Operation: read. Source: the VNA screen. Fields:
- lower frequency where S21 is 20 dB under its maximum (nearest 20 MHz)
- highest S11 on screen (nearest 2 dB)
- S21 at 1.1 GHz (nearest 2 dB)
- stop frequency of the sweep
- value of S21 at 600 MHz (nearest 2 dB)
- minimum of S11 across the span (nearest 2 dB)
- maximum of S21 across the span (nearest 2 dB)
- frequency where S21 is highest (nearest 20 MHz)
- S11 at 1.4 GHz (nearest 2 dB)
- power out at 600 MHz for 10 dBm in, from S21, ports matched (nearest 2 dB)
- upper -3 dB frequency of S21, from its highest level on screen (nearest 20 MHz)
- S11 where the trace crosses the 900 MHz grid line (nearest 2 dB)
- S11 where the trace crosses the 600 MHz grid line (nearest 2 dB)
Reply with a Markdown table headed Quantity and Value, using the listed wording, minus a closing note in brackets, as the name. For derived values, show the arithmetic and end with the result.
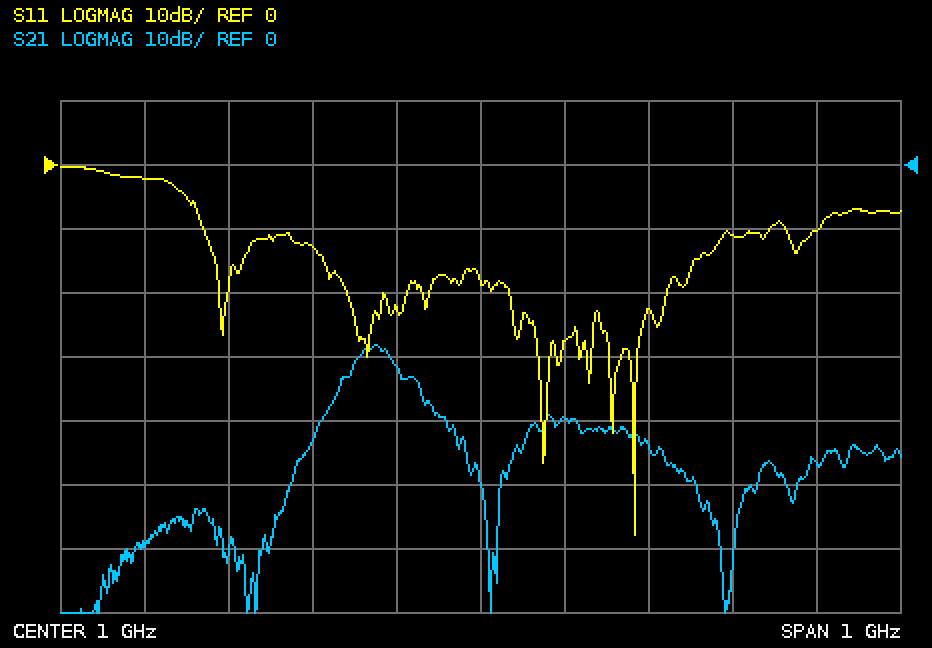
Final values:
| Quantity | Value |
|---|---|
| lower frequency where S21 is 20 dB under its maximum | 780 MHz |
| highest S11 on screen | 0 dB |
| S21 at 1.1 GHz | -40 dB |
| stop frequency of the sweep | 1.5 GHz |
| value of S21 at 600 MHz | -60 dB |
| minimum of S11 across the span | -58 dB |
| maximum of S21 across the span | -28 dB |
| frequency where S21 is highest | 880 MHz |
| S11 at 1.4 GHz | -10 dB |
| power out at 600 MHz for 10 dBm in, from S21, ports matched | 10 dBm + (-60 dB) = -50 dBm |
| upper -3 dB frequency of S21, from its highest level on screen | 900 MHz |
| S11 where the trace crosses the 900 MHz grid line | -22 dB |
| S11 where the trace crosses the 600 MHz grid line | -2 dB |
